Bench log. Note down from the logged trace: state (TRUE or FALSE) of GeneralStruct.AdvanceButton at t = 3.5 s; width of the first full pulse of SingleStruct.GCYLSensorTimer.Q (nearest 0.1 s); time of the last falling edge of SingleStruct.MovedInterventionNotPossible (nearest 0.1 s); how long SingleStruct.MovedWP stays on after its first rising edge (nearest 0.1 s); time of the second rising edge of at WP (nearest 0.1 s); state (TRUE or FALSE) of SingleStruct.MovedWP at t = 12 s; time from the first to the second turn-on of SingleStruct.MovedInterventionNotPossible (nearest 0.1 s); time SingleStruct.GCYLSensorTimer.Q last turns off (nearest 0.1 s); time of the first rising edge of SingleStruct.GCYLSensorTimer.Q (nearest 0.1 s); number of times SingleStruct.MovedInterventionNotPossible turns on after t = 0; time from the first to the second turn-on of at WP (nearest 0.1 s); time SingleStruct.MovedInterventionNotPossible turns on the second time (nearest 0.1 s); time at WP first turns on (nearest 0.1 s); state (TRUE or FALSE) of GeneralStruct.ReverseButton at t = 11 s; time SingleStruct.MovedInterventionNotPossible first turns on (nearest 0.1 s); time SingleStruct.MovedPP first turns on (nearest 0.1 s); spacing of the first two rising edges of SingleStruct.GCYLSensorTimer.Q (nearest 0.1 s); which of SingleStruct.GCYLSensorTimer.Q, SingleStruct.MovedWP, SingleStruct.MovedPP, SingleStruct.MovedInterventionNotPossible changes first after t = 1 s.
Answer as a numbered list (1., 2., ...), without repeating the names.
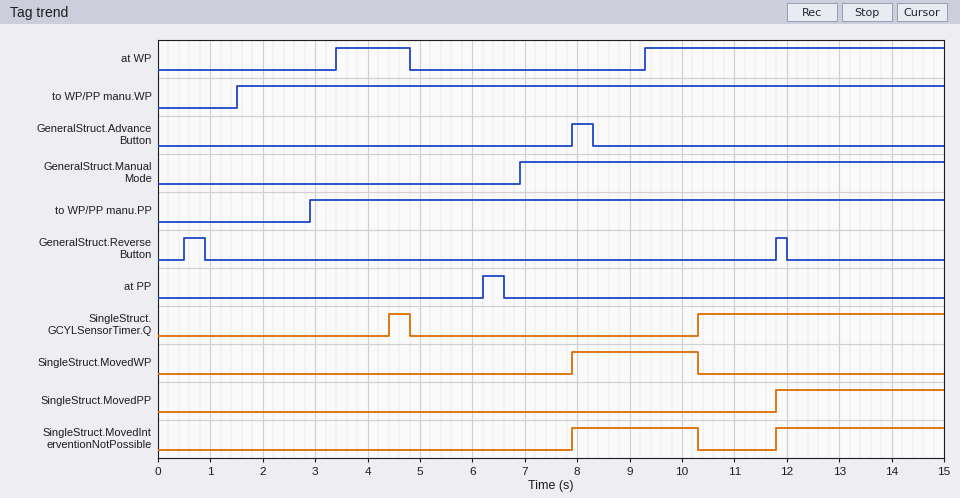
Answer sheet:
1. FALSE
2. 0.4 s
3. 10.3 s
4. 2.4 s
5. 9.3 s
6. FALSE
7. 3.9 s
8. 4.8 s
9. 4.4 s
10. 2
11. 5.9 s
12. 11.8 s
13. 3.4 s
14. FALSE
15. 7.9 s
16. 11.8 s
17. 5.9 s
18. SingleStruct.GCYLSensorTimer.Q
